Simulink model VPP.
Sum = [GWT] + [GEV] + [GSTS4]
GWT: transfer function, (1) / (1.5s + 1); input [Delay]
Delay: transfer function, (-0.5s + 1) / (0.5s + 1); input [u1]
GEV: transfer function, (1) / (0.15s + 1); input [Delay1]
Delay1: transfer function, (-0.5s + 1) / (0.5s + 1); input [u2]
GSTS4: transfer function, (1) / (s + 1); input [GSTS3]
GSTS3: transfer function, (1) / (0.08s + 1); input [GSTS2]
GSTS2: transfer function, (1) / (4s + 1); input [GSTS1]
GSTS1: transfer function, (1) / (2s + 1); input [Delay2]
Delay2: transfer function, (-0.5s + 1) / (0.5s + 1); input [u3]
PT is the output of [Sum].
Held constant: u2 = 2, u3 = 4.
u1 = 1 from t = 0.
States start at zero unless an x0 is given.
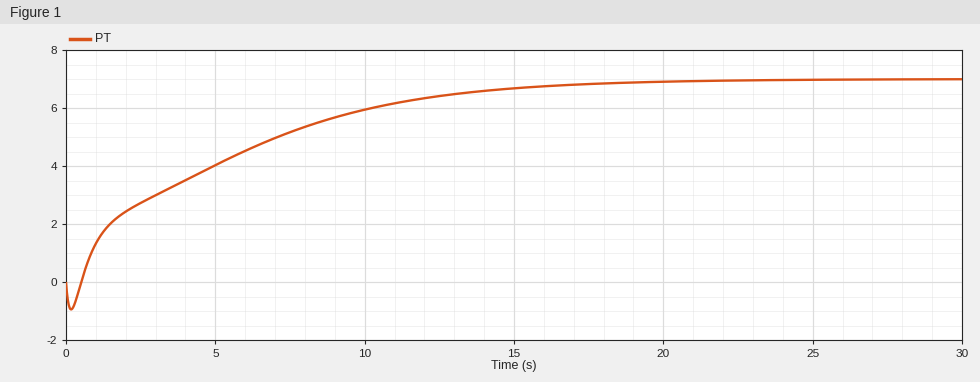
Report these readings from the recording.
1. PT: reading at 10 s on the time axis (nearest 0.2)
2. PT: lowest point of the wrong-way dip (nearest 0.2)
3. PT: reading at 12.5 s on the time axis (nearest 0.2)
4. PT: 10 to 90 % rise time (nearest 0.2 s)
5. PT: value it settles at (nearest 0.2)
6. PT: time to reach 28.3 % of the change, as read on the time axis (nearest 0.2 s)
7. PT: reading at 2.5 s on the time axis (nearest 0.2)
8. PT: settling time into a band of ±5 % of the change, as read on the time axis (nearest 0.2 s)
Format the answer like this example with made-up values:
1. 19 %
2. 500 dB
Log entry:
1. 6.0
2. -1.0
3. 6.4
4. 11.0 s
5. 7.0
6. 1.4 s
7. 2.8
8. 14.6 s
